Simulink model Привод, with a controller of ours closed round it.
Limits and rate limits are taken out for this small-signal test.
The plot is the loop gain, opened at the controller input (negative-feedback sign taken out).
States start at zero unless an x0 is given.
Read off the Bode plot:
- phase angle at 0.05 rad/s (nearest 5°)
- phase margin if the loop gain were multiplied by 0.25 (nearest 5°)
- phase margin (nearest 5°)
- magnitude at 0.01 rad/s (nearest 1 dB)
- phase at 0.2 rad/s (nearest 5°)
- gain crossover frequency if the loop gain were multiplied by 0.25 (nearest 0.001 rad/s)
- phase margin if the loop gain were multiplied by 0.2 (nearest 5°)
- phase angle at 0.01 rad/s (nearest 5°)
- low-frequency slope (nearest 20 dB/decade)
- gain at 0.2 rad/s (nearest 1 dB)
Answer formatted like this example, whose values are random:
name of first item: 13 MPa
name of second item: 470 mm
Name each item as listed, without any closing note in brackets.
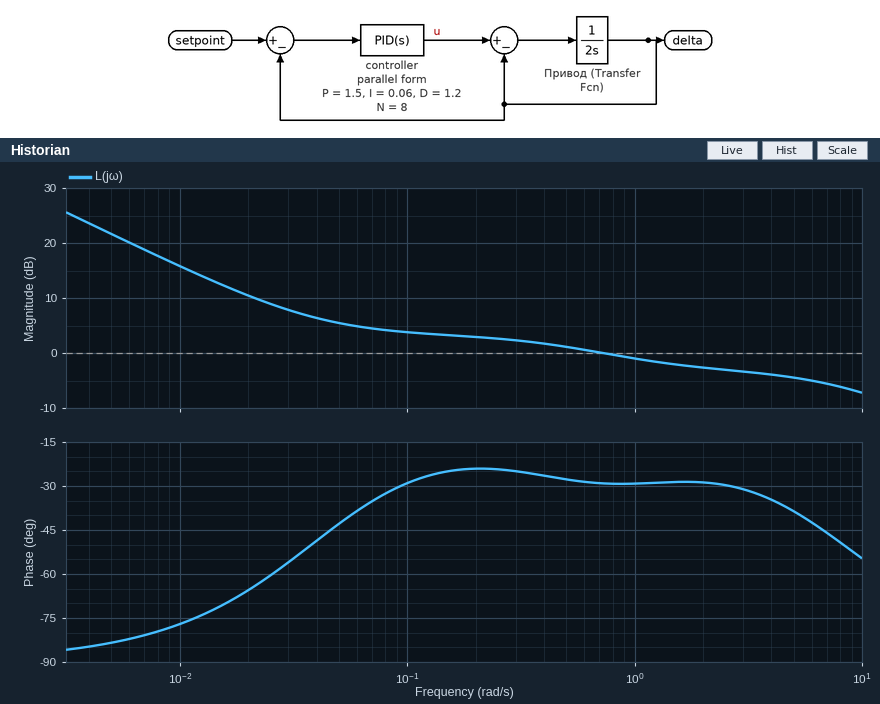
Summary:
phase angle at 0.05 rad/s: -45°
phase margin if the loop gain were multiplied by 0.25: 110°
phase margin: 150°
magnitude at 0.01 rad/s: 16 dB
phase at 0.2 rad/s: -25°
gain crossover frequency if the loop gain were multiplied by 0.25: 0.016 rad/s
phase margin if the loop gain were multiplied by 0.2: 105°
phase angle at 0.01 rad/s: -75°
low-frequency slope: -20 dB/decade
gain at 0.2 rad/s: 3 dB
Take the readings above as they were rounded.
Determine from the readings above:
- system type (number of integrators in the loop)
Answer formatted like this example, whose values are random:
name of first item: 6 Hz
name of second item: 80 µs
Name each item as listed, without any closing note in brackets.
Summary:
system type: 1
